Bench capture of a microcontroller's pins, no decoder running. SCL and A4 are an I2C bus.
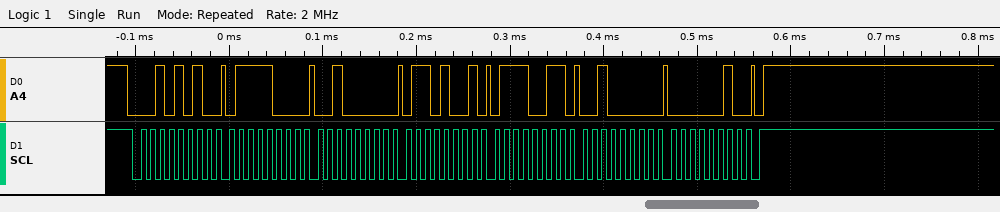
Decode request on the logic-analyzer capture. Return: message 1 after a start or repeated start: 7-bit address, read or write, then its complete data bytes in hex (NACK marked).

0x15 write: 78 20 69 73 20 02
